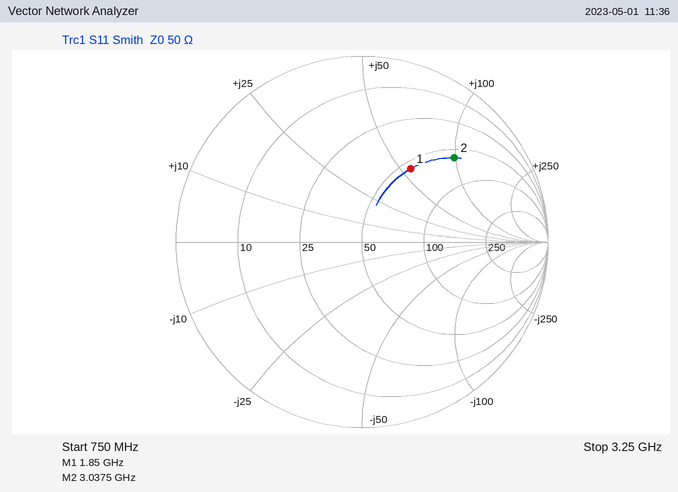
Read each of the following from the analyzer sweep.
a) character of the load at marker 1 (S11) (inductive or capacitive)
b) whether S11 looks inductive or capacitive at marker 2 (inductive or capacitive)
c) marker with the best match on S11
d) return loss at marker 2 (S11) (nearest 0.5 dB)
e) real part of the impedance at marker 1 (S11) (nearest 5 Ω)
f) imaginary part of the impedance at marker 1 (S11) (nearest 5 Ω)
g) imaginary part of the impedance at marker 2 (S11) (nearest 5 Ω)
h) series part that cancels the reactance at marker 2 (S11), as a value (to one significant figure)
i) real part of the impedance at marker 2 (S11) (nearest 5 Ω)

inductive
inductive
marker 1
3.5 dB
55 Ω
+55 Ω
+100 Ω
500 fF
60 Ω
